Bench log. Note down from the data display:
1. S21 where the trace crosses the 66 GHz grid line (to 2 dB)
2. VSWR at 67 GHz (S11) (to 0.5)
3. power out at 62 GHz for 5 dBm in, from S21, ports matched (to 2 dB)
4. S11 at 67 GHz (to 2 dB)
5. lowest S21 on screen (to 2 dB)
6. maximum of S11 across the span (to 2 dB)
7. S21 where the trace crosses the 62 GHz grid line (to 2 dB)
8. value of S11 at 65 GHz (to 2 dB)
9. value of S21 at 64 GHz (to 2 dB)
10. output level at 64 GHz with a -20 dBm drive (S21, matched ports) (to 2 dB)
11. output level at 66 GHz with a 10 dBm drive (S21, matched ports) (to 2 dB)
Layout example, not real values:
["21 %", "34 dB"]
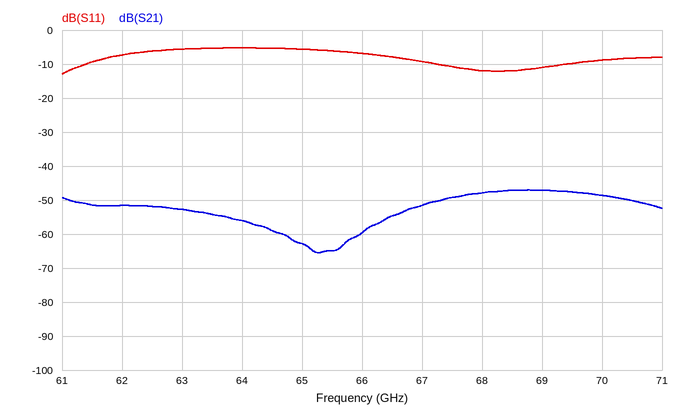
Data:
["-60 dB", "2.0", "-46 dBm", "-10 dB", "-66 dB", "-6 dB", "-52 dB", "-6 dB", "-56 dB", "-76 dBm", "-50 dBm"]
